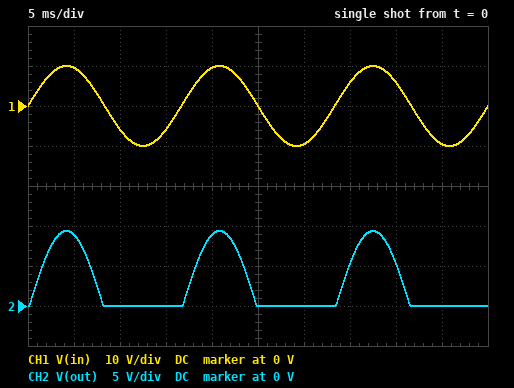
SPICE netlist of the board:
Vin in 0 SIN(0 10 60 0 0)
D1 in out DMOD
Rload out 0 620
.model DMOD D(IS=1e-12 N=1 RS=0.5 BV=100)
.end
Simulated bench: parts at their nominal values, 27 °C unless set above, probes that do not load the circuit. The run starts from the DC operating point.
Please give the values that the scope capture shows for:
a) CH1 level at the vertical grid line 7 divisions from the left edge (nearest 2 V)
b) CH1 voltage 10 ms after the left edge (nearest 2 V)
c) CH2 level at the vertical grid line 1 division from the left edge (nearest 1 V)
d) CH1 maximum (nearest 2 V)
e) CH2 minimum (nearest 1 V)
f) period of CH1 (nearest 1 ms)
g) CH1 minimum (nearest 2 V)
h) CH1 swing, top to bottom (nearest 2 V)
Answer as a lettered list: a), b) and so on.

a) 6 V
b) -6 V
c) 9 V
d) 10 V
e) 0 V
f) 17 ms
g) -10 V
h) 20 V
